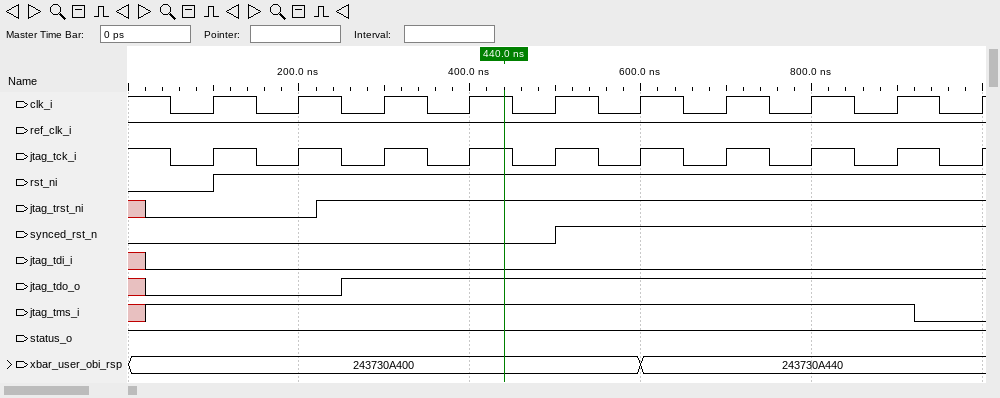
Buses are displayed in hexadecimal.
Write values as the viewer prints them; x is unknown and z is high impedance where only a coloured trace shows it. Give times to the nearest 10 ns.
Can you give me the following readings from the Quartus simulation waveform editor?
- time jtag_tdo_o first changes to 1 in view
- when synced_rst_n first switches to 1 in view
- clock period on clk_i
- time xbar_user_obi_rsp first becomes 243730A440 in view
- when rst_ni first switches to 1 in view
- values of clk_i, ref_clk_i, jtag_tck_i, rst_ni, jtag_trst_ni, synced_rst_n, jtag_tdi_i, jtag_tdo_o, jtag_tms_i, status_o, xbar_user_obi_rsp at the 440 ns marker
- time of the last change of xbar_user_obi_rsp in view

250 ns
500 ns
100 ns
600 ns
100 ns
clk_i=1, ref_clk_i=1, jtag_tck_i=1, rst_ni=1, jtag_trst_ni=1, synced_rst_n=0, jtag_tdi_i=0, jtag_tdo_o=1, jtag_tms_i=1, status_o=1, xbar_user_obi_rsp=243730A400
600 ns
